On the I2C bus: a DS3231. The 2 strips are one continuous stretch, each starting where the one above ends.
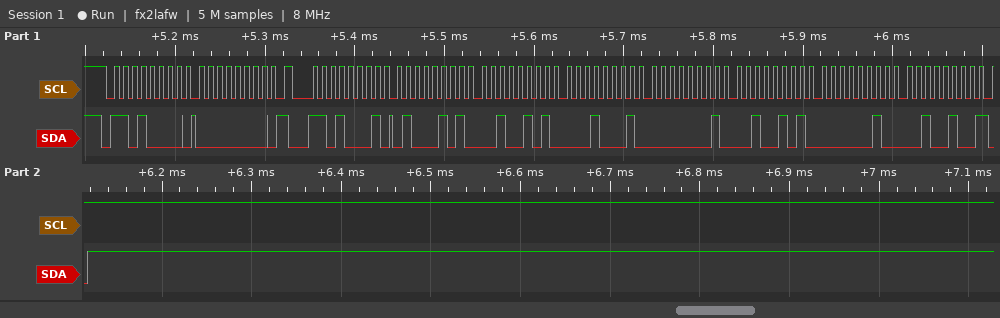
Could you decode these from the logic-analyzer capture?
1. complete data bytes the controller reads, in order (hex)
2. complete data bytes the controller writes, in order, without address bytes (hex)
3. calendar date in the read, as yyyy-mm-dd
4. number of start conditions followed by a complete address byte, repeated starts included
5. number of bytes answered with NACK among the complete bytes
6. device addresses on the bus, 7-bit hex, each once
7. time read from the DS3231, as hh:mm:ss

45 25 11 01 25 02 24
00
2024-02-25
2
1
0x68
11:25:45
